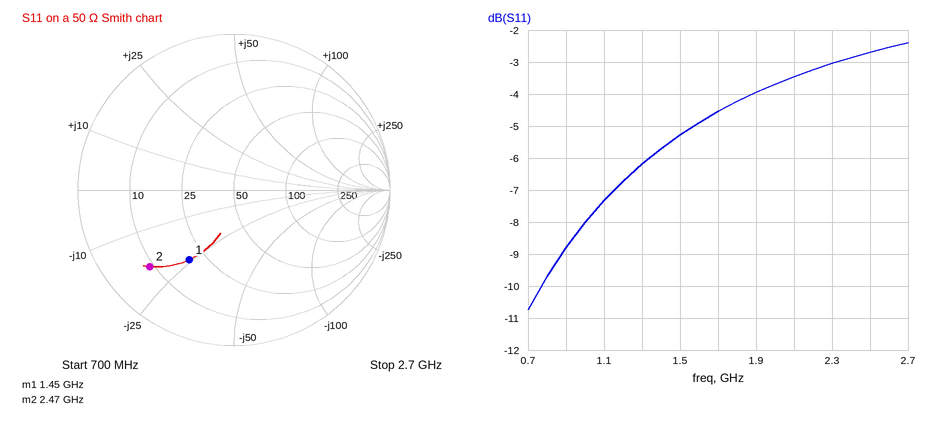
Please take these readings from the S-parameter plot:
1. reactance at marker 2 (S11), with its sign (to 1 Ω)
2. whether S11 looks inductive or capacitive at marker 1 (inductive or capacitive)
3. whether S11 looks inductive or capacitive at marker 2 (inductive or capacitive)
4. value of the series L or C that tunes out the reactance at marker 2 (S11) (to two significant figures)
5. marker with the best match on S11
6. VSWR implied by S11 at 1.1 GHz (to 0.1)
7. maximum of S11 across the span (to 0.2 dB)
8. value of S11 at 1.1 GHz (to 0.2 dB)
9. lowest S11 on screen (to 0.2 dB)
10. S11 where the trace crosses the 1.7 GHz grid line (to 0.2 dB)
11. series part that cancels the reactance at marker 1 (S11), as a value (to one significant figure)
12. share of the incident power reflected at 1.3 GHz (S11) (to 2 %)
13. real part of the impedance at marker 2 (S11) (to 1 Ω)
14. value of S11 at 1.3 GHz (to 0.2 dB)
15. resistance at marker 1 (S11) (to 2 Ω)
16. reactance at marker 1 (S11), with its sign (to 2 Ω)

-19 Ω
capacitive
capacitive
1.2 nH
marker 1
2.5
-2.4 dB
-7.4 dB
-10.8 dB
-4.6 dB
3 nH
24 %
9 Ω
-6.2 dB
20 Ω
-24 Ω
